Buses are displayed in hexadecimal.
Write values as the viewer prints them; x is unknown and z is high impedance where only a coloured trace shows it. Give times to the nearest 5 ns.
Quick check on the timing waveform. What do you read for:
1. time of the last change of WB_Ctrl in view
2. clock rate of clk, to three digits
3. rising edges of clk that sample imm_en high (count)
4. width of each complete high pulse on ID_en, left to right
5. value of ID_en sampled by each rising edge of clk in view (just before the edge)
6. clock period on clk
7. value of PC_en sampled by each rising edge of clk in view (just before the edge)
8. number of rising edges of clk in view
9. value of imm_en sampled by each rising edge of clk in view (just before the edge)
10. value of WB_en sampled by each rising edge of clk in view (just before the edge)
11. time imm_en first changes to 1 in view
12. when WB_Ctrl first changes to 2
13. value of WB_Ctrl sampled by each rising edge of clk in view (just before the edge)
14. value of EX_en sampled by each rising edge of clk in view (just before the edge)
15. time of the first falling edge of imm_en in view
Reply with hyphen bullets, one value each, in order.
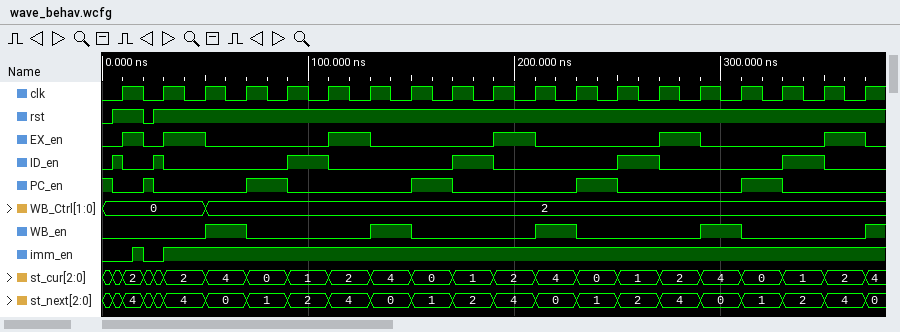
- 50 ns
- 50.0 MHz
- 17
- 5 ns, 5 ns, 20 ns, 20 ns, 20 ns, 20 ns
- 1 1 0 0 0 1 0 0 0 1 0 0 0 1 0 0 0 1 0
- 20 ns
- 0 0 0 0 1 0 0 0 1 0 0 0 1 0 0 0 1 0 0
- 19
- 0 0 1 1 1 1 1 1 1 1 1 1 1 1 1 1 1 1 1
- 0 0 0 1 0 0 0 1 0 0 0 1 0 0 0 1 0 0 0
- 15 ns
- 50 ns
- 0, 0, 0, 2, 2, 2, 2, 2, 2, 2, 2, 2, 2, 2, 2, 2, 2, 2, 2
- 0 0 1 0 0 0 1 0 0 0 1 0 0 0 1 0 0 0 1
- 20 ns
